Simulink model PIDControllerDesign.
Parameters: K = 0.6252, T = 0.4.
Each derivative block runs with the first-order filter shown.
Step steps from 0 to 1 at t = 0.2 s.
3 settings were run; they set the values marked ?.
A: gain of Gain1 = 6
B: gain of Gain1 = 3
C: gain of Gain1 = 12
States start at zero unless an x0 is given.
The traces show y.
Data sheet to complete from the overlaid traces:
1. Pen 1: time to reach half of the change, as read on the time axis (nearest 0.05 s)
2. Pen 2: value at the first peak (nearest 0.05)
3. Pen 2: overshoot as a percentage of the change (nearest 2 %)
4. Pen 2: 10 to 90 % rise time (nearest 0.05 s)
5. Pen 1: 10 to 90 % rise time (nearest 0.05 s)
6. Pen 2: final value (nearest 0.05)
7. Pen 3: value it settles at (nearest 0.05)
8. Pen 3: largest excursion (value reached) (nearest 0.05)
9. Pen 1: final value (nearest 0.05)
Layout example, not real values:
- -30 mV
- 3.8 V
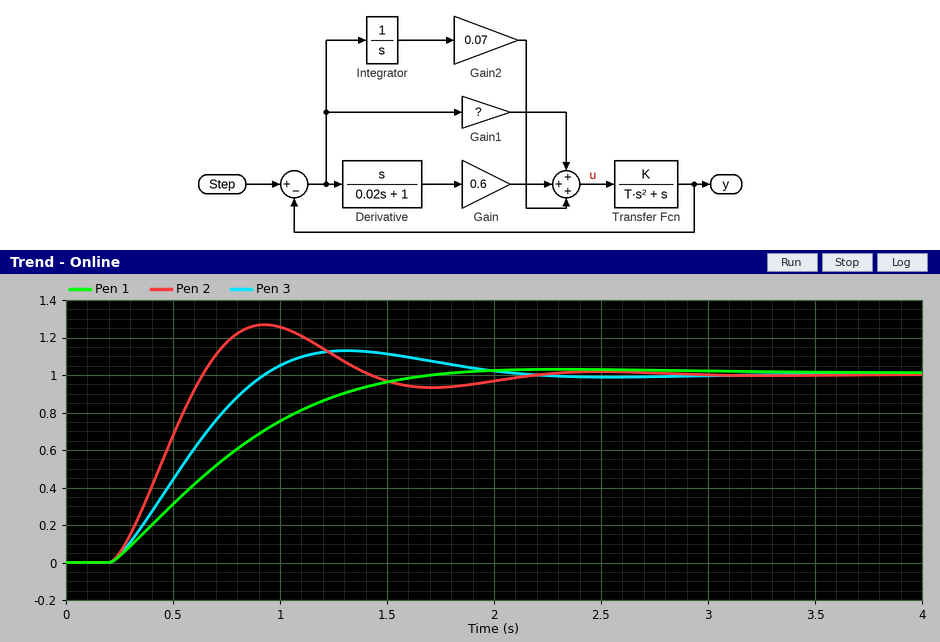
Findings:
- 0.70 s
- 1.25
- 26 %
- 0.30 s
- 1.00 s
- 1.00
- 1.00
- 1.15
- 1.00
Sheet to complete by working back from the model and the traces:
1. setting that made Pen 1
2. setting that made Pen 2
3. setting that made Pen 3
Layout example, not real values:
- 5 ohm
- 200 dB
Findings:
- B
- C
- A
